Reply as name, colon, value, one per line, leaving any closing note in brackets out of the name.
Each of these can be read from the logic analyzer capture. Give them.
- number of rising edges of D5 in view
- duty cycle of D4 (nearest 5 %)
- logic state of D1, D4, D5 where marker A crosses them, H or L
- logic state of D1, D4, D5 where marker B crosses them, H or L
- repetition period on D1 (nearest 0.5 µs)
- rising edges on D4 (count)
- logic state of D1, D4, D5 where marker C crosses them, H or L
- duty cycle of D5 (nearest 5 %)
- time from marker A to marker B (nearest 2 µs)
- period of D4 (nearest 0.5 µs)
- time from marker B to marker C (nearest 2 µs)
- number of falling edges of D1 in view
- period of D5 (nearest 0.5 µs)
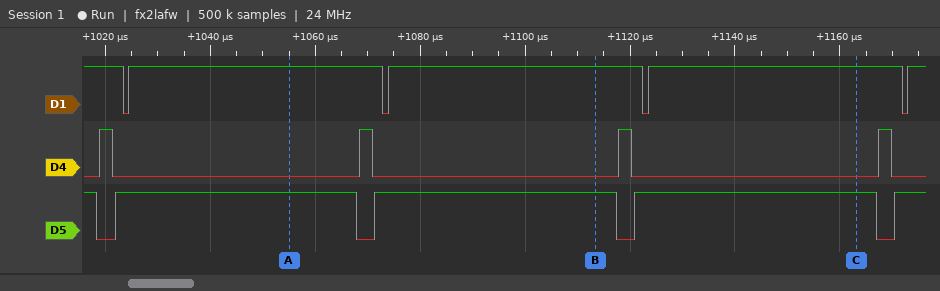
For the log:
number of rising edges of D5 in view: 4
duty cycle of D4: 5 %
logic state of D1, D4, D5 where marker A crosses them, H or L: D1=H, D4=L, D5=H
logic state of D1, D4, D5 where marker B crosses them, H or L: D1=H, D4=L, D5=H
repetition period on D1: 49.5 µs
rising edges on D4: 4
logic state of D1, D4, D5 where marker C crosses them, H or L: D1=H, D4=L, D5=H
duty cycle of D5: 95 %
time from marker A to marker B: 58 µs
period of D4: 49.5 µs
time from marker B to marker C: 50 µs
number of falling edges of D1 in view: 4
period of D5: 49.5 µs
